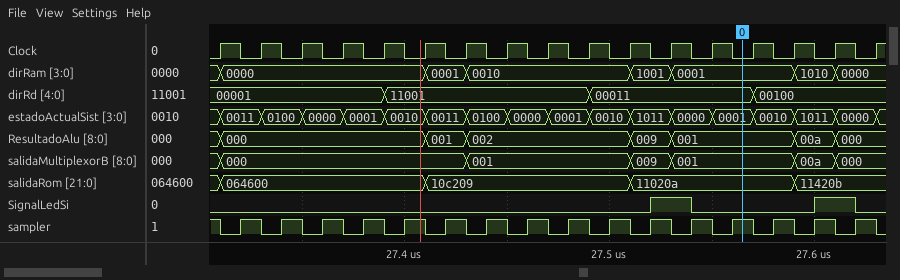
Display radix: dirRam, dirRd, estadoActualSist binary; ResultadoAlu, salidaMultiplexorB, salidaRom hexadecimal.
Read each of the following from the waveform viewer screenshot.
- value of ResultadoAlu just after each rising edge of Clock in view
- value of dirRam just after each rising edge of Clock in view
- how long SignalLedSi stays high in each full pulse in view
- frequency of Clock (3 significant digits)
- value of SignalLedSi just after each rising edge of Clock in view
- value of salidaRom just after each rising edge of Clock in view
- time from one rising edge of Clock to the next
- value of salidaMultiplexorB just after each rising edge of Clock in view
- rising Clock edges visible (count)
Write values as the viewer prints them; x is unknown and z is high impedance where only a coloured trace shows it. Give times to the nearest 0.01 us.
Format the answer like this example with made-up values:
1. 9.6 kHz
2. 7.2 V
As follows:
1. 000, 000, 000, 000, 000, 001, 002, 002, 002, 002, 009, 001, 001, 001, 00a, 000, 000
2. 0000, 0000, 0000, 0000, 0000, 0001, 0010, 0010, 0010, 0010, 1001, 0001, 0001, 0001, 1010, 0000, 0000
3. 0.02 us, 0.02 us
4. 50.0 MHz
5. 0 0 0 0 0 0 0 0 0 0 0 1 0 0 0 1 0
6. 064600, 064600, 064600, 064600, 064600, 10c209, 10c209, 10c209, 10c209, 10c209, 11020a, 11020a, 11020a, 11020a, 11420b, 11420b, 11420b
7. 0.02 us
8. 000, 000, 000, 000, 000, 000, 001, 001, 001, 001, 009, 001, 001, 001, 00a, 000, 000
9. 17
